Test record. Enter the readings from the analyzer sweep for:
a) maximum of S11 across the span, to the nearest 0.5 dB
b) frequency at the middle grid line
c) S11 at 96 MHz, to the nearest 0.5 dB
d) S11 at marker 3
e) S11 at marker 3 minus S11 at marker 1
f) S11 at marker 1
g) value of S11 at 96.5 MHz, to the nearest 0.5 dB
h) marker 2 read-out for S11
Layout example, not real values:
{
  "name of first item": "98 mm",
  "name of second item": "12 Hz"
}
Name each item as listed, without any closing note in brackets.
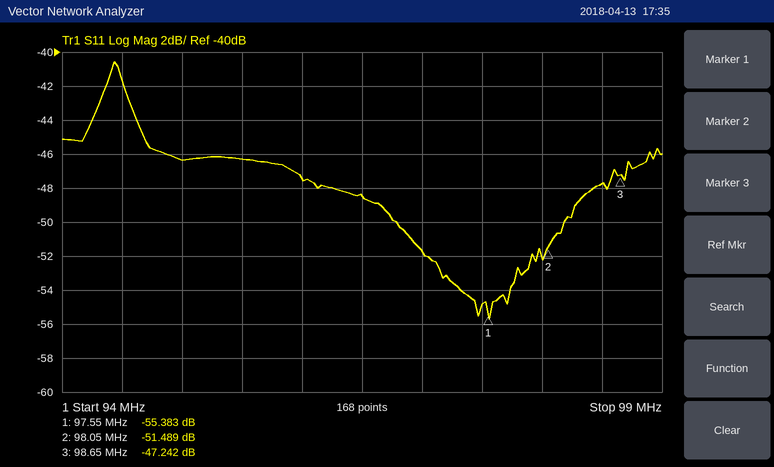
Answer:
{
  "maximum of S11 across the span, to the nearest 0.5 dB": "-40.5 dB",
  "frequency at the middle grid line": "96.5 MHz",
  "S11 at 96 MHz, to the nearest 0.5 dB": "-47.5 dB",
  "S11 at marker 3": "-47.242 dB",
  "S11 at marker 3 minus S11 at marker 1": "8.141 dB",
  "S11 at marker 1": "-55.383 dB",
  "value of S11 at 96.5 MHz, to the nearest 0.5 dB": "-48.5 dB",
  "marker 2 read-out for S11": "-51.489 dB"
}
